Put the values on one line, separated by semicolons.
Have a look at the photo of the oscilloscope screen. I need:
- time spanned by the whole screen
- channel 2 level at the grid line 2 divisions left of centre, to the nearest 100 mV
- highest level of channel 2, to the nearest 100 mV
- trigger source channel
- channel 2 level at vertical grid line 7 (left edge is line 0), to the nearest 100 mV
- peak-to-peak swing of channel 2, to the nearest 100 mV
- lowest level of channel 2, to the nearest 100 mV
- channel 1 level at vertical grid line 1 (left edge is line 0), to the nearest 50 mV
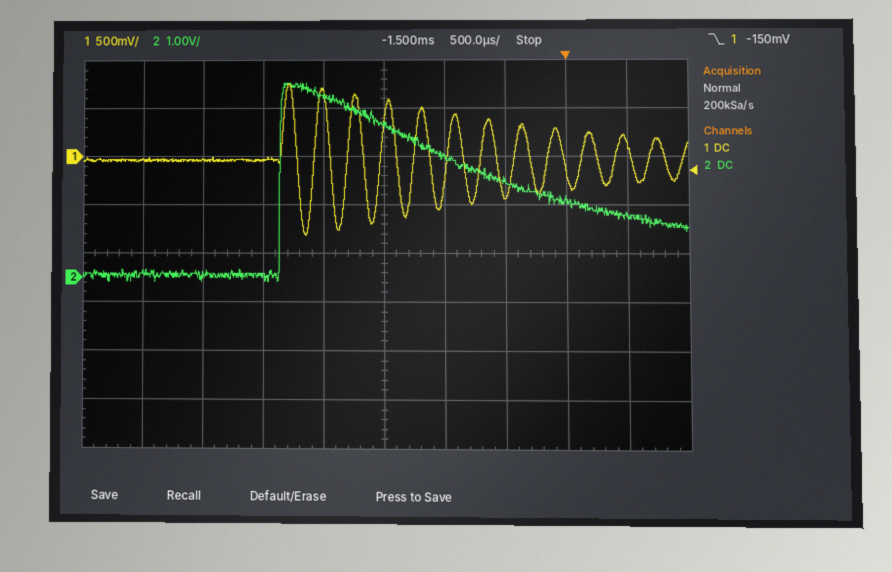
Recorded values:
5 ms; 0.0 V; 4.0 V; channel 1; 2.0 V; 4.1 V; -100 mV; -50 mV
